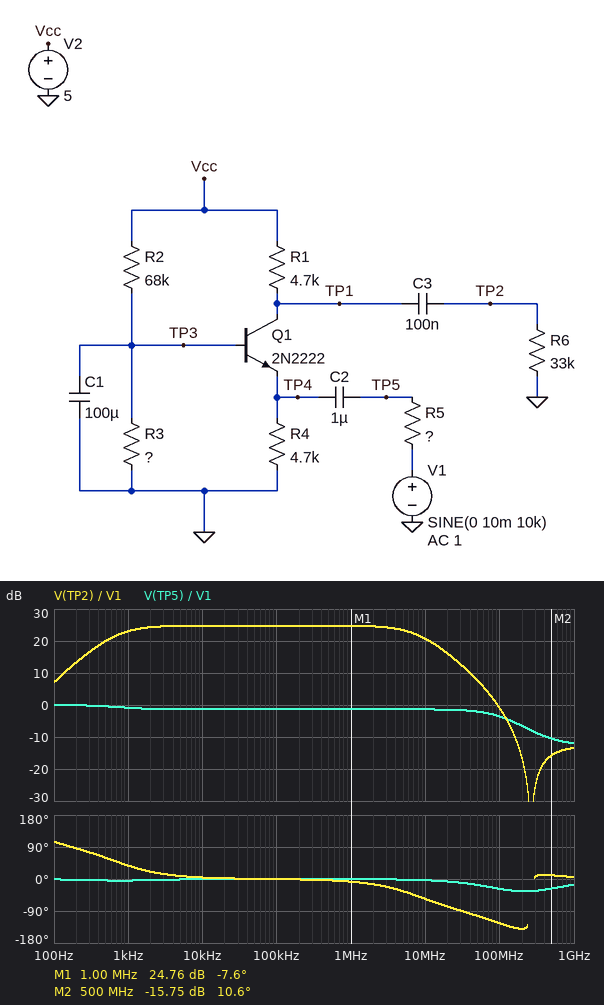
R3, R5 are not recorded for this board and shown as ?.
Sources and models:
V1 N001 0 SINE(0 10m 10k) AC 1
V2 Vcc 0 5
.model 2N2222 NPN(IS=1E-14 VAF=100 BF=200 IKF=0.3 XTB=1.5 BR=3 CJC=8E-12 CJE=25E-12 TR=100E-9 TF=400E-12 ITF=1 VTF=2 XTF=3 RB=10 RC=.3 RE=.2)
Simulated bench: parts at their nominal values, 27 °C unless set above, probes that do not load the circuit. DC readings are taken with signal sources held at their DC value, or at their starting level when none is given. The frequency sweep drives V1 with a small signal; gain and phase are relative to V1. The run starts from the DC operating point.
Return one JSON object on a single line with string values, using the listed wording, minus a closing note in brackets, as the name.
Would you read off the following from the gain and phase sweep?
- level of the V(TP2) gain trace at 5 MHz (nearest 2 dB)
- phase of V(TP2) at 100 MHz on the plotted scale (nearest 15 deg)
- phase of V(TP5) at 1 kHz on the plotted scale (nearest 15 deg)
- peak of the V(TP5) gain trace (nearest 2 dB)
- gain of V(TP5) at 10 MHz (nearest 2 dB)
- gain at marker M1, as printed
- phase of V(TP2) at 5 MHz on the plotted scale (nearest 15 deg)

{"level of the V(TP2) gain trace at 5 MHz": "24 dB", "phase of V(TP2) at 100 MHz on the plotted scale": "-120 deg", "phase of V(TP5) at 1 kHz on the plotted scale": "0 deg", "peak of the V(TP5) gain trace": "0 dB", "gain of V(TP5) at 10 MHz": "-2 dB", "gain at marker M1, as printed": "24.76 dB", "phase of V(TP2) at 5 MHz on the plotted scale": "-30 deg"}
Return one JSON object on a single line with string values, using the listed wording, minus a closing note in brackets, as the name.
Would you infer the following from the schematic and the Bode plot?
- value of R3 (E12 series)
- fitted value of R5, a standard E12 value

{"value of R3": "22 kΩ", "fitted value of R5, a standard E12 value": "33 Ω"}
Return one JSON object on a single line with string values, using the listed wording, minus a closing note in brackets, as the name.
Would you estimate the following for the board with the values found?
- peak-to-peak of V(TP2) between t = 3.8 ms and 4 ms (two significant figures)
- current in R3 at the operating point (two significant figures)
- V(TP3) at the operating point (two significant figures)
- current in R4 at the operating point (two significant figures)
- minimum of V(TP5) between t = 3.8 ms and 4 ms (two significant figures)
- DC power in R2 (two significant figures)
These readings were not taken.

{"peak-to-peak of V(TP2) between t = 3.8 ms and 4 ms": "340 mV", "current in R3 at the operating point": "55 µA", "V(TP3) at the operating point": "1.2 V", "current in R4 at the operating point": "130 µA", "minimum of V(TP5) between t = 3.8 ms and 4 ms": "-8.5 mV", "DC power in R2": "210 µW"}
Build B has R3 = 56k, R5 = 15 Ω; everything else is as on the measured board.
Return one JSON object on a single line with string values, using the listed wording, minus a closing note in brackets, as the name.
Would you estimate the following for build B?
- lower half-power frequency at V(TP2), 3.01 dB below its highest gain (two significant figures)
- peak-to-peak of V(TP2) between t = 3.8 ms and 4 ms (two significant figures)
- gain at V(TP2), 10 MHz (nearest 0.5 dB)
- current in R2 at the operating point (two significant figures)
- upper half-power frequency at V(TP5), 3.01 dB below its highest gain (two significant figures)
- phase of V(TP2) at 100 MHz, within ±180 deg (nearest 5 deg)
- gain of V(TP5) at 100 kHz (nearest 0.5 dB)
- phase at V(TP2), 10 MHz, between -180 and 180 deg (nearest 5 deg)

{"lower half-power frequency at V(TP2), 3.01 dB below its highest gain": "1.7 kHz", "peak-to-peak of V(TP2) between t = 3.8 ms and 4 ms": "850 mV", "gain at V(TP2), 10 MHz": "27.0 dB", "current in R2 at the operating point": "41 µA", "upper half-power frequency at V(TP5), 3.01 dB below its highest gain": "160 MHz", "phase of V(TP2) at 100 MHz, within ±180 deg": "-110 deg", "gain of V(TP5) at 100 kHz": "-1.5 dB", "phase at V(TP2), 10 MHz, between -180 and 180 deg": "-60 deg"}
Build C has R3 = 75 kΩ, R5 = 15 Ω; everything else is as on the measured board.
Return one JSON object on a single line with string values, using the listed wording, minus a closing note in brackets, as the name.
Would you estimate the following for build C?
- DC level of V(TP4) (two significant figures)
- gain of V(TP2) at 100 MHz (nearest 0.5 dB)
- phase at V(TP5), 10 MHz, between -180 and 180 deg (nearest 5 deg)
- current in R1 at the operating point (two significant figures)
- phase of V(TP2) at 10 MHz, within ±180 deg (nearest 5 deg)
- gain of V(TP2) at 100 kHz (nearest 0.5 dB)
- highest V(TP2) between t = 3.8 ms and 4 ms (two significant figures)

{"DC level of V(TP4)": "1.9 V", "gain of V(TP2) at 100 MHz": "7.0 dB", "phase at V(TP5), 10 MHz, between -180 and 180 deg": "0 deg", "current in R1 at the operating point": "410 µA", "phase of V(TP2) at 10 MHz, within ±180 deg": "-65 deg", "gain of V(TP2) at 100 kHz": "34.0 dB", "highest V(TP2) between t = 3.8 ms and 4 ms": "470 mV"}
